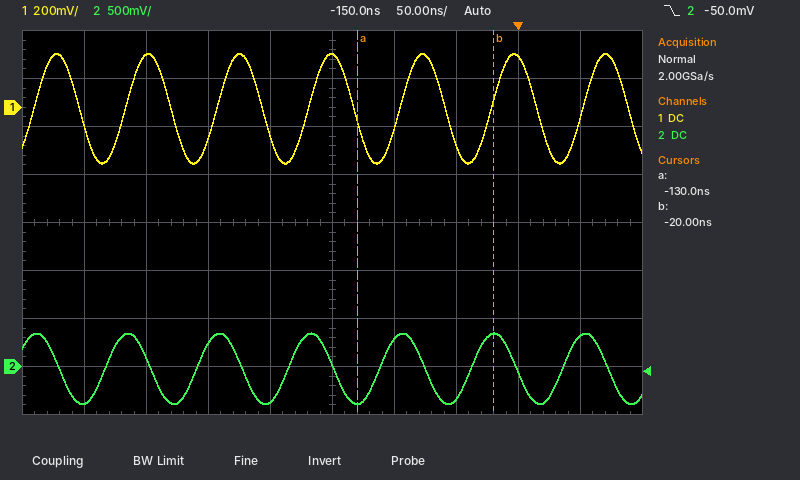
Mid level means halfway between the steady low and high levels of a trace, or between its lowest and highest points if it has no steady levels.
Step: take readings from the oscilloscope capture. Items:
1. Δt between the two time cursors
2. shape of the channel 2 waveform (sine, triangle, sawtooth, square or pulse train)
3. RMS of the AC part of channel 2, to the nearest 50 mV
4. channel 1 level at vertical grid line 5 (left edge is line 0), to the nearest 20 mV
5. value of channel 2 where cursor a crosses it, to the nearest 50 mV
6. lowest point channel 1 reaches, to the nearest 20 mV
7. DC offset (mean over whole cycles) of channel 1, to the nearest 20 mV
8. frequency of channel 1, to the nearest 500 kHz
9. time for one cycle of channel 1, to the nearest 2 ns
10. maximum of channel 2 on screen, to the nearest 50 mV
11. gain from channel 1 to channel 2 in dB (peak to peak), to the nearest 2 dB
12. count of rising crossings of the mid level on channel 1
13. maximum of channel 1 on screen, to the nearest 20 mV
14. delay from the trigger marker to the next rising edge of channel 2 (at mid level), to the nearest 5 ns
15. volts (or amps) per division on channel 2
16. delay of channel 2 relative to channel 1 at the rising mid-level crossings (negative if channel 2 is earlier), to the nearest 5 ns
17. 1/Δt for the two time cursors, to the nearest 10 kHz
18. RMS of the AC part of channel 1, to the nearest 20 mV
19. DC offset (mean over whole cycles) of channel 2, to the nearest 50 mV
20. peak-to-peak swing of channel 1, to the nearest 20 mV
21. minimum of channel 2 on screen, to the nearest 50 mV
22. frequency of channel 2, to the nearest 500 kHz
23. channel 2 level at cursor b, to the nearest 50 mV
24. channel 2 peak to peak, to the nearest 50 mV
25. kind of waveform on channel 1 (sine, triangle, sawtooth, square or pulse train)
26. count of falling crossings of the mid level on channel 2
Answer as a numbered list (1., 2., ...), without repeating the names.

1. 110 ns
2. sine
3. 250 mV
4. 220 mV
5. -400 mV
6. -240 mV
7. 0 mV
8. 13.5 MHz
9. 74 ns
10. 350 mV
11. 4 dB
12. 7
13. 220 mV
14. 35 ns
15. 500 mV
16. -15 ns
17. 9.09 MHz
18. 160 mV
19. 0 mV
20. 460 mV
21. -400 mV
22. 13.5 MHz
23. 350 mV
24. 750 mV
25. sine
26. 7
